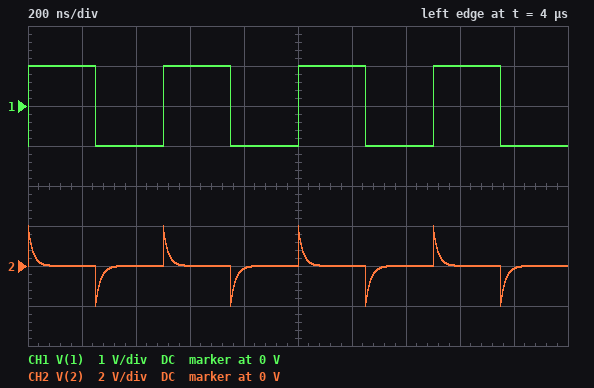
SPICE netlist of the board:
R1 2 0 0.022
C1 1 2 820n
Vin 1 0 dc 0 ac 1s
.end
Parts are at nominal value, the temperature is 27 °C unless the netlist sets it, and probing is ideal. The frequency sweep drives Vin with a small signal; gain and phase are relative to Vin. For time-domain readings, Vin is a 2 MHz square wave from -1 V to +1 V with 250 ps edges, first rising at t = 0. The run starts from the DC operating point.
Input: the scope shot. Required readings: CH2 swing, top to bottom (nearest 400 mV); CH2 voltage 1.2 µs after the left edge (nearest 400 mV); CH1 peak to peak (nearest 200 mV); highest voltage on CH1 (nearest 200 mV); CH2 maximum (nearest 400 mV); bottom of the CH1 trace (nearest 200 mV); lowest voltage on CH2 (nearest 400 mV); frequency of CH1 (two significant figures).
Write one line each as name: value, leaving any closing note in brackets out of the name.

CH2 swing, top to bottom: 4.0 V
CH2 voltage 1.2 µs after the left edge: 0 V
CH1 peak to peak: 2.0 V
highest voltage on CH1: 1.0 V
CH2 maximum: 2.0 V
bottom of the CH1 trace: -1.0 V
lowest voltage on CH2: -2.0 V
frequency of CH1: 2.0 MHz
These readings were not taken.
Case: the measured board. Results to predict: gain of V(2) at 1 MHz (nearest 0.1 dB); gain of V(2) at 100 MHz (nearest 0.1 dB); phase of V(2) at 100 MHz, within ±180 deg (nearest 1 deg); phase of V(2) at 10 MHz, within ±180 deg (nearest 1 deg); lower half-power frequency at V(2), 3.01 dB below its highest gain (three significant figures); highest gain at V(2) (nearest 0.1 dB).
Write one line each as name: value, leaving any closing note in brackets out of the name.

gain of V(2) at 1 MHz: -19.0 dB
gain of V(2) at 100 MHz: 0 dB
phase of V(2) at 100 MHz, within ±180 deg: 5 deg
phase of V(2) at 10 MHz, within ±180 deg: 41 deg
lower half-power frequency at V(2), 3.01 dB below its highest gain: 8.82 MHz
highest gain at V(2): 0 dB
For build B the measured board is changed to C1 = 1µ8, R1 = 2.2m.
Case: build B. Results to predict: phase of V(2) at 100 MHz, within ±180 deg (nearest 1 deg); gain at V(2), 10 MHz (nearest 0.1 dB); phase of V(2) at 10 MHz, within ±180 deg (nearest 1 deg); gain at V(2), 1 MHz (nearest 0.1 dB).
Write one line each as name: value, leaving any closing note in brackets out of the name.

phase of V(2) at 100 MHz, within ±180 deg: 22 deg
gain at V(2), 10 MHz: -12.3 dB
phase of V(2) at 10 MHz, within ±180 deg: 76 deg
gain at V(2), 1 MHz: -32.1 dB
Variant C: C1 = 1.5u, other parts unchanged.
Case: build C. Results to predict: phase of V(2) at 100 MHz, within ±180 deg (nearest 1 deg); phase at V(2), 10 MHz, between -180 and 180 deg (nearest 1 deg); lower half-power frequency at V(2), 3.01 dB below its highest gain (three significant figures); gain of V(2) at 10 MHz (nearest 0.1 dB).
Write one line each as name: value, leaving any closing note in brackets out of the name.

phase of V(2) at 100 MHz, within ±180 deg: 3 deg
phase at V(2), 10 MHz, between -180 and 180 deg: 26 deg
lower half-power frequency at V(2), 3.01 dB below its highest gain: 4.82 MHz
gain of V(2) at 10 MHz: -0.9 dB
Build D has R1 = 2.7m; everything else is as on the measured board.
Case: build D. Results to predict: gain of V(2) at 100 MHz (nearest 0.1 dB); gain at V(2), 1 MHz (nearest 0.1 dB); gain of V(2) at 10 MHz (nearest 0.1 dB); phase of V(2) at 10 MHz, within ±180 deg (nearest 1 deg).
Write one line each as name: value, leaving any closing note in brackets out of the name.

gain of V(2) at 100 MHz: -1.8 dB
gain at V(2), 1 MHz: -37.1 dB
gain of V(2) at 10 MHz: -17.2 dB
phase of V(2) at 10 MHz, within ±180 deg: 82 deg
